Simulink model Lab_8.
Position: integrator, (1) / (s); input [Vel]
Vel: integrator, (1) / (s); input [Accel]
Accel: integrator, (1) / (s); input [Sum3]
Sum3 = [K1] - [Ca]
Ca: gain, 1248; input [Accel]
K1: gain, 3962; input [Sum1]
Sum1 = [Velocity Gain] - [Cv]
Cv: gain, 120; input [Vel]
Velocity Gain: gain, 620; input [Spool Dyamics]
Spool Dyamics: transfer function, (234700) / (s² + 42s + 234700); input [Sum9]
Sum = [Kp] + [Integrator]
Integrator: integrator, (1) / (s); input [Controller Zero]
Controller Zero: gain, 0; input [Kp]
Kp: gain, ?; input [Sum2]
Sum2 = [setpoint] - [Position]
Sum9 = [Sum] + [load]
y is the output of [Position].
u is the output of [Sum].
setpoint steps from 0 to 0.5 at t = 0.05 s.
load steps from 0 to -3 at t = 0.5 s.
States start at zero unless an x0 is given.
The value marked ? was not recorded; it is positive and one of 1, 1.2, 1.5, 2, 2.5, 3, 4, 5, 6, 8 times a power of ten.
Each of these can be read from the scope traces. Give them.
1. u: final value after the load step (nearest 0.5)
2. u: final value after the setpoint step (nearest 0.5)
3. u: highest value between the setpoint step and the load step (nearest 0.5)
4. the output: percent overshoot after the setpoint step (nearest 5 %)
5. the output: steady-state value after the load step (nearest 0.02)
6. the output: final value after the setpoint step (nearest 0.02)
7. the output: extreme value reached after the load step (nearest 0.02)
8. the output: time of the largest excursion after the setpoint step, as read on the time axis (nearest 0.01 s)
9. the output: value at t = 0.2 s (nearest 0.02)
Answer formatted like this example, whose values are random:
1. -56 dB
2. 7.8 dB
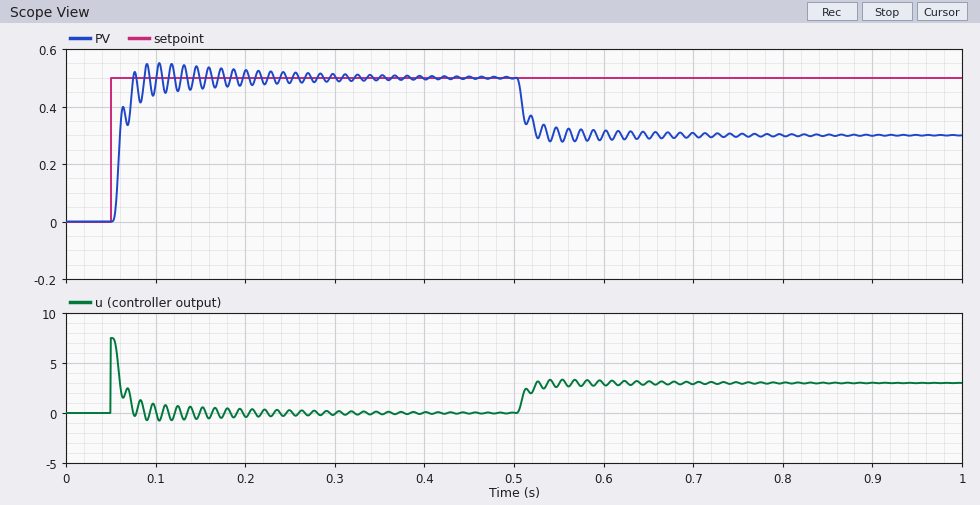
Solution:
1. 3.0
2. 0.0
3. 7.5
4. 10 %
5. 0.30
6. 0.50
7. 0.28
8. 0.10 s
9. 0.52
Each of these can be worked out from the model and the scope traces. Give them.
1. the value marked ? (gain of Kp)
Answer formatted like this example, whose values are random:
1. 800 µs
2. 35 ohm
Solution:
1. 15
